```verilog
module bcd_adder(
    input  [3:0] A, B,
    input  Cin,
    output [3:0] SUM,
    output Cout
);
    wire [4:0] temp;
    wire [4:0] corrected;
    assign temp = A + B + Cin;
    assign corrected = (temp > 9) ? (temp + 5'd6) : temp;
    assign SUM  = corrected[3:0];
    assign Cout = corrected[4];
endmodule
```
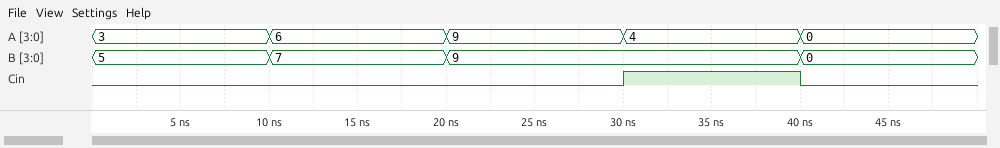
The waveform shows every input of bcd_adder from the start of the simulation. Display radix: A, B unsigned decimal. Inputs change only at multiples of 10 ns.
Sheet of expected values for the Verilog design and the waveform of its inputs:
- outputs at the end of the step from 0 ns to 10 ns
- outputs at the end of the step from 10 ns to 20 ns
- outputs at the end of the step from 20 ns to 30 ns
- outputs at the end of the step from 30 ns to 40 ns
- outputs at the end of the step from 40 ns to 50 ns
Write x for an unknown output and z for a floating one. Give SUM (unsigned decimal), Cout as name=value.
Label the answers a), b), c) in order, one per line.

a) SUM=8, Cout=0
b) SUM=3, Cout=1
c) SUM=8, Cout=1
d) SUM=4, Cout=1
e) SUM=0, Cout=0
